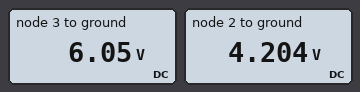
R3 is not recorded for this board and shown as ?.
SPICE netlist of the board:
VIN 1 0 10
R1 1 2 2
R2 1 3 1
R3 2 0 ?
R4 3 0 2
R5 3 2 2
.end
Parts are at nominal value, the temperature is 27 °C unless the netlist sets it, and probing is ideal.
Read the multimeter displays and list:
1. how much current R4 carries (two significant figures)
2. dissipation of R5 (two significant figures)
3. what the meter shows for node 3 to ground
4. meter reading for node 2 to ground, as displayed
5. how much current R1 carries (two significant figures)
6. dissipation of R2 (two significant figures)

3.0 A
1.7 W
6.05 V
4.204 V
2.9 A
16 W
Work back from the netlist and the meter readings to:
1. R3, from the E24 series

1.1 Ω
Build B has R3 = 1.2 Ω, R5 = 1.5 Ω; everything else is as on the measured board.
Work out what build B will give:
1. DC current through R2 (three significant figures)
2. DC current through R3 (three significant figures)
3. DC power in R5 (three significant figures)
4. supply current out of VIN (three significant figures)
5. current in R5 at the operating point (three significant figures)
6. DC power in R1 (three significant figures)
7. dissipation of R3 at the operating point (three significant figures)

4.00 A
3.75 A
1.50 W
6.75 A
1.00 A
15.1 W
16.9 W
